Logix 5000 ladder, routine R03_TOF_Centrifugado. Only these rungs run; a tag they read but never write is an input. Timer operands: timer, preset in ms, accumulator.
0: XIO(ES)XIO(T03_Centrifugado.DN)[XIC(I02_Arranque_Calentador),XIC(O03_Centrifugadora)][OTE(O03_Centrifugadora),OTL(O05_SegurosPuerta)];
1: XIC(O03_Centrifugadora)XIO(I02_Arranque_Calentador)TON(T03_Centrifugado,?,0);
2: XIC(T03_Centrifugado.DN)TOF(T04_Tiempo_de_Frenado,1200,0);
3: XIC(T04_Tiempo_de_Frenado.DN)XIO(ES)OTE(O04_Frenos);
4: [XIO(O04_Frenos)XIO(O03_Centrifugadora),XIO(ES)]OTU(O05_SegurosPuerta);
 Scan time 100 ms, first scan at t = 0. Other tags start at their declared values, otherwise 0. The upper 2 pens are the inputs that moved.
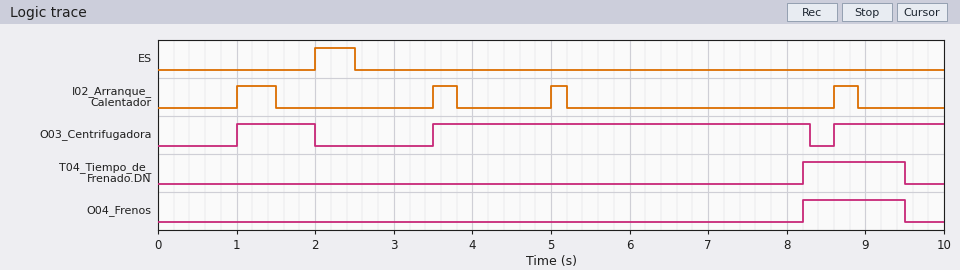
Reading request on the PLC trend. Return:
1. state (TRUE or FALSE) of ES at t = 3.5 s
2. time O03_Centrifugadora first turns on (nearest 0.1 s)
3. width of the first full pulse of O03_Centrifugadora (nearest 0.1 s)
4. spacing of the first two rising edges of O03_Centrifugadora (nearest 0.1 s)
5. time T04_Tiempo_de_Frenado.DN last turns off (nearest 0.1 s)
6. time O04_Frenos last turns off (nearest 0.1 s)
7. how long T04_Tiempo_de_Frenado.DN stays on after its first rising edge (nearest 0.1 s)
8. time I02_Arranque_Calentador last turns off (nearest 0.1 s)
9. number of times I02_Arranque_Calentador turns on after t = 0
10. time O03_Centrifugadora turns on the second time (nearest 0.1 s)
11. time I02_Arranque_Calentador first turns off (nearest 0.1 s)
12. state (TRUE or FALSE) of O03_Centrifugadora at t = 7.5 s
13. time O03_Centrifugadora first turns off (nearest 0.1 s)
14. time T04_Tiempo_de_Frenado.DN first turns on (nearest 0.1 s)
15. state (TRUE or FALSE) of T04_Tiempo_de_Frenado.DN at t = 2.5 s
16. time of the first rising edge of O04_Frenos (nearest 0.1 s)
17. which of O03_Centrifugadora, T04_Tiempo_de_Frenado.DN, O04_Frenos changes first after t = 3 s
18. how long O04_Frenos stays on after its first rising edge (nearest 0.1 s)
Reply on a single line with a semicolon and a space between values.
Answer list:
FALSE; 1.0 s; 1.0 s; 2.5 s; 9.5 s; 9.5 s; 1.3 s; 8.9 s; 4; 3.5 s; 1.5 s; TRUE; 2.0 s; 8.2 s; FALSE; 8.2 s; O03_Centrifugadora; 1.3 s
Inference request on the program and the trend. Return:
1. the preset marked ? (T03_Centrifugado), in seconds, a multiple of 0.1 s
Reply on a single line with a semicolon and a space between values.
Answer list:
3.0 s
